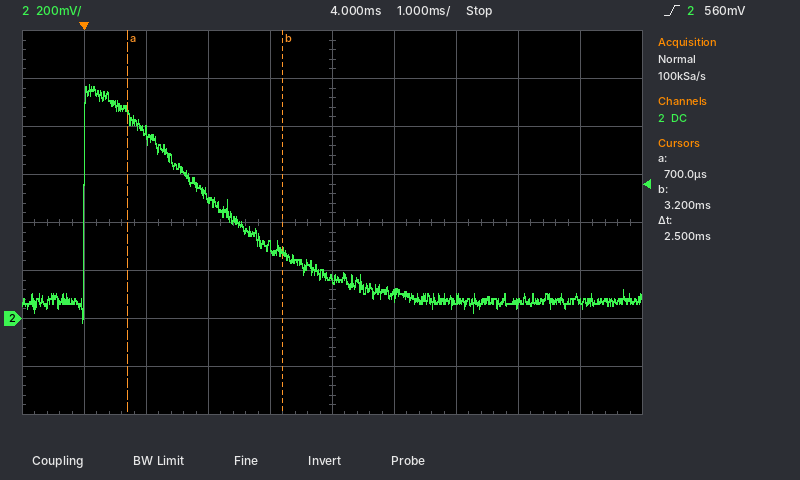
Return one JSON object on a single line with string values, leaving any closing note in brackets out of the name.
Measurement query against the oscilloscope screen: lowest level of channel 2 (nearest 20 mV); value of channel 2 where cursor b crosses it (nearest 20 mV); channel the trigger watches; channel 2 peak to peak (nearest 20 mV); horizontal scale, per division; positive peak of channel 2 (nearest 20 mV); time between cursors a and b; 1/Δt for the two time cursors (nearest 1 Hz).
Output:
{"lowest level of channel 2": "-20 mV", "value of channel 2 where cursor b crosses it": "280 mV", "channel the trigger watches": "channel 2", "channel 2 peak to peak": "1.00 V", "horizontal scale, per division": "1 ms", "positive peak of channel 2": "980 mV", "time between cursors a and b": "2.5 ms", "1/Δt for the two time cursors": "400 Hz"}
